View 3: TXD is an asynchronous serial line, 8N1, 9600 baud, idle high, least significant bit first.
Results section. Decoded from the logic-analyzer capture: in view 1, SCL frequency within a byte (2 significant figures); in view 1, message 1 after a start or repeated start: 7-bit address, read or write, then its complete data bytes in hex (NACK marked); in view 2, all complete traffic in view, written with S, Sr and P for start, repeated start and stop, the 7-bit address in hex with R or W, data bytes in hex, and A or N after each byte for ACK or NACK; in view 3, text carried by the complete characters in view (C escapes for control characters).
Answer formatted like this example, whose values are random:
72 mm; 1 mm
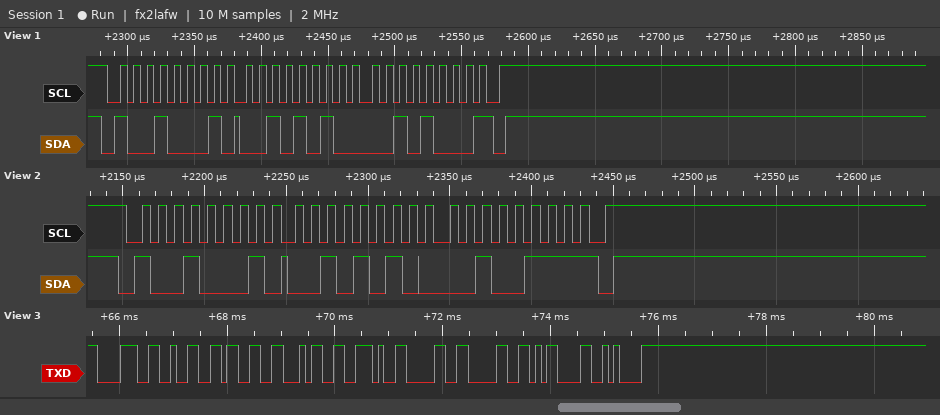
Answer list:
100 kHz; 0x48 read: 2A 28 NACK; S 48R A 2A A 27 N P; "8234.00\r\n"
